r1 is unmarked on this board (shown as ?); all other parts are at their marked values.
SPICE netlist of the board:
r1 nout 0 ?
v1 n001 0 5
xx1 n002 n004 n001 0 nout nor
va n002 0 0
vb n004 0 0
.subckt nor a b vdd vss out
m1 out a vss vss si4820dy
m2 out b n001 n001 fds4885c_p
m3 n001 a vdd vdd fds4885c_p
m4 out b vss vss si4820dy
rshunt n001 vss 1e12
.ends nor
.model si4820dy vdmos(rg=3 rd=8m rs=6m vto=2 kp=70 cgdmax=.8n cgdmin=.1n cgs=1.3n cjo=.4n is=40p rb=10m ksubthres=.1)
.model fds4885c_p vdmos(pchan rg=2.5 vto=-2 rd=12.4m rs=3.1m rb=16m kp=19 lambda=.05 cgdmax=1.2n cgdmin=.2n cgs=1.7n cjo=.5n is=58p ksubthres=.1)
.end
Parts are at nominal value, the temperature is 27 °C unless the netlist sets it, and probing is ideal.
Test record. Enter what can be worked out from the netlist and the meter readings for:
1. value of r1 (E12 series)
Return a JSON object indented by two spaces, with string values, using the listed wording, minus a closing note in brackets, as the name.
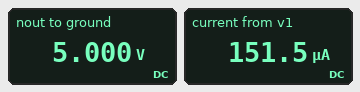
{
  "value of r1": "33 kΩ"
}
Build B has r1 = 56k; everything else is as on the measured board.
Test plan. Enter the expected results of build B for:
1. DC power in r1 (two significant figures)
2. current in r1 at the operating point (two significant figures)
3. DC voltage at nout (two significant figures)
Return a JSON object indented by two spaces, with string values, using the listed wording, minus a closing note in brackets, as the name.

{
  "DC power in r1": "450 µW",
  "current in r1 at the operating point": "89 µA",
  "DC voltage at nout": "5.0 V"
}
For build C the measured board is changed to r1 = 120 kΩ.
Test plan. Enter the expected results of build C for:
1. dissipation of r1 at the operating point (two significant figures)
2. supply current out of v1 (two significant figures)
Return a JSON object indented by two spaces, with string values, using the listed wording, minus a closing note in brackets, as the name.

{
  "dissipation of r1 at the operating point": "210 µW",
  "supply current out of v1": "42 µA"
}
